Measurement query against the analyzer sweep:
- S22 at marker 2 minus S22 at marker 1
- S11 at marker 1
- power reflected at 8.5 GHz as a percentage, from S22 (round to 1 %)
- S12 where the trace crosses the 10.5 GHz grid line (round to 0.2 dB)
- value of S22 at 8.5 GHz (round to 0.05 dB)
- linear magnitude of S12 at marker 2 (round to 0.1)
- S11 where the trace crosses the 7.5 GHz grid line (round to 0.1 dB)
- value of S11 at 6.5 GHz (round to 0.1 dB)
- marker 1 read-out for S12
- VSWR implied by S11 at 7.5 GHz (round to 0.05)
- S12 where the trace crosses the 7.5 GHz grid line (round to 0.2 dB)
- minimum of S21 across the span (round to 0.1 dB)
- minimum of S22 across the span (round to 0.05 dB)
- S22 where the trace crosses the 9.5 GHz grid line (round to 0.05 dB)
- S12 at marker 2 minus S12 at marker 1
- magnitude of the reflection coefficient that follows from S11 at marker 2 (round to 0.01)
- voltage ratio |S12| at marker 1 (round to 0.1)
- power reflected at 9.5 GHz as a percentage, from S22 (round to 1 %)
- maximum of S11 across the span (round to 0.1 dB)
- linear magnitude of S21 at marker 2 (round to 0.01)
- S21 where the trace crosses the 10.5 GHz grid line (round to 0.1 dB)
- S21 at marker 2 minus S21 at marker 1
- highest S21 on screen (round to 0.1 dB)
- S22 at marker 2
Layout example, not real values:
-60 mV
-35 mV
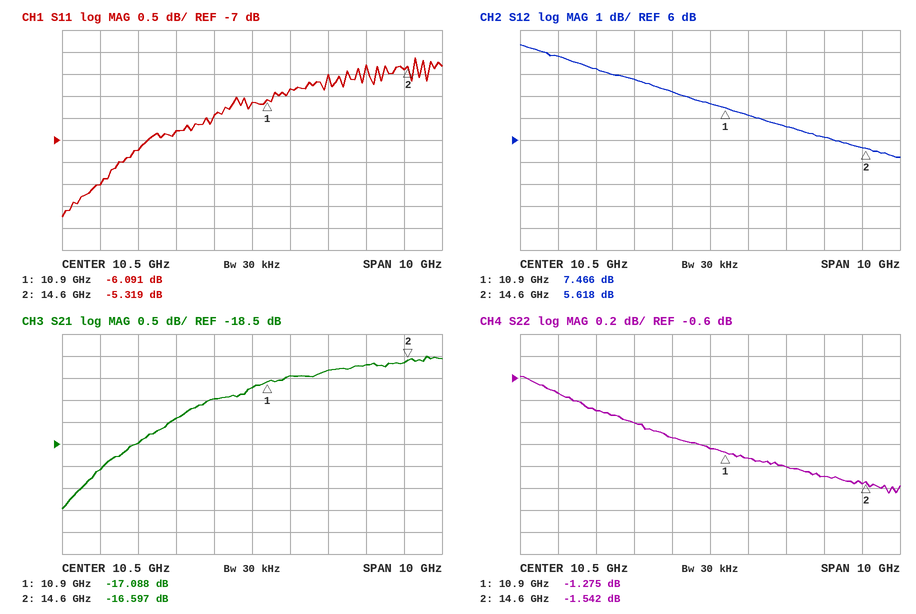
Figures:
-0.267 dB
-6.091 dB
79 %
7.6 dB
-1.00 dB
1.9
-7.2 dB
-8.0 dB
7.466 dB
2.55
9.2 dB
-20.0 dB
-1.65 dB
-1.15 dB
-1.848 dB
0.54
2.4
77 %
-5.1 dB
0.15
-17.2 dB
0.491 dB
-16.5 dB
-1.542 dB
